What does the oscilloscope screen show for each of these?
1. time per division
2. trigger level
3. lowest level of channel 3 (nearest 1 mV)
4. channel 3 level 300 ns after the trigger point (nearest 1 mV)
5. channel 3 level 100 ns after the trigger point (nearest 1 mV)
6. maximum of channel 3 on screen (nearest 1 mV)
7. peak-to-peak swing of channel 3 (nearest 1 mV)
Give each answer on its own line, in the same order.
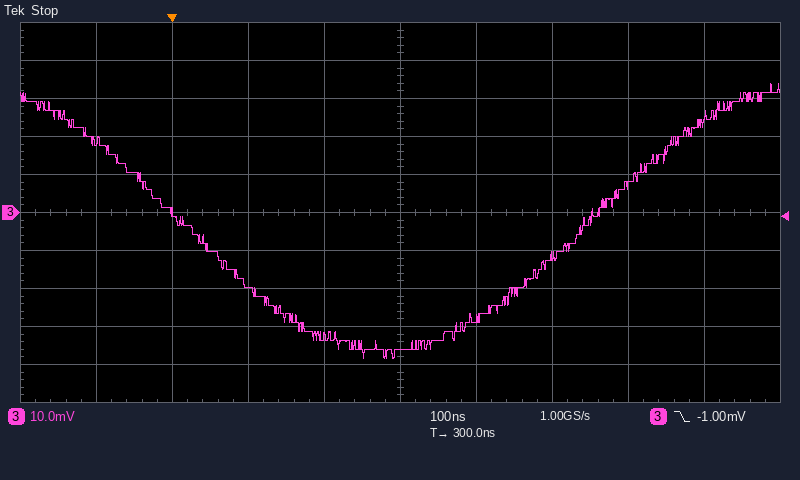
100 ns
-1.00 mV
-38 mV
-36 mV
-19 mV
34 mV
72 mV
